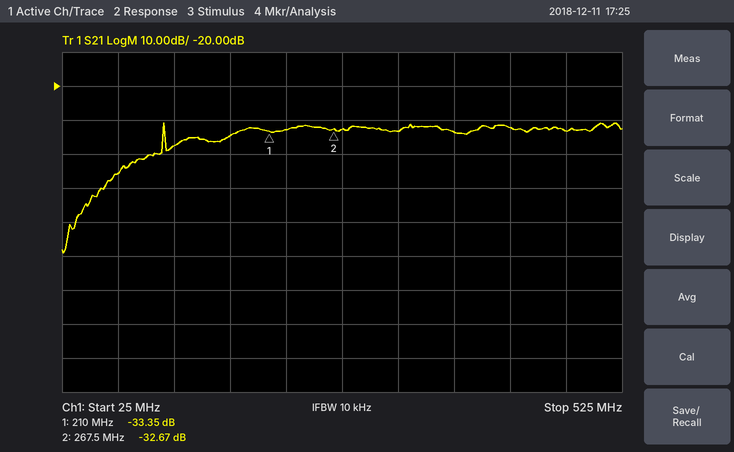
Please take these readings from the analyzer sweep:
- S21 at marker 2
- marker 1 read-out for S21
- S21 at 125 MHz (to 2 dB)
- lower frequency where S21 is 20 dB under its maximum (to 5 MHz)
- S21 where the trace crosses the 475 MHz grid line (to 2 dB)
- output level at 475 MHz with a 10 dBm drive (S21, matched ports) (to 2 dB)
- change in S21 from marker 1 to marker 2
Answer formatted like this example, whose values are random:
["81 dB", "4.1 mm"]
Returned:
["-32.67 dB", "-33.35 dB", "-38 dB", "60 MHz", "-34 dB", "-24 dBm", "0.68 dB"]
